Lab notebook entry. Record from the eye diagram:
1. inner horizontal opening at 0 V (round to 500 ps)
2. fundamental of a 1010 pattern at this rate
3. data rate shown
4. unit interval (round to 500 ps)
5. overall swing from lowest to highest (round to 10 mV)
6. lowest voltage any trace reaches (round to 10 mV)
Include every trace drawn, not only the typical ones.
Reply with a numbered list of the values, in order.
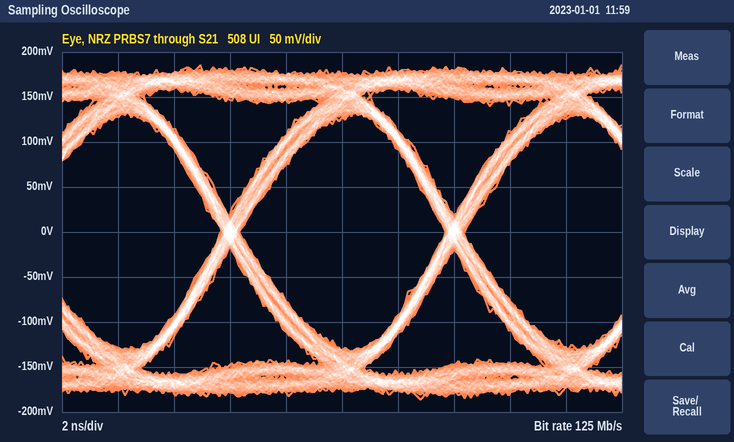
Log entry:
1. 7.5 ns
2. 62.5 MHz
3. 125 Mb/s
4. 8.0 ns
5. 370 mV
6. -190 mV
